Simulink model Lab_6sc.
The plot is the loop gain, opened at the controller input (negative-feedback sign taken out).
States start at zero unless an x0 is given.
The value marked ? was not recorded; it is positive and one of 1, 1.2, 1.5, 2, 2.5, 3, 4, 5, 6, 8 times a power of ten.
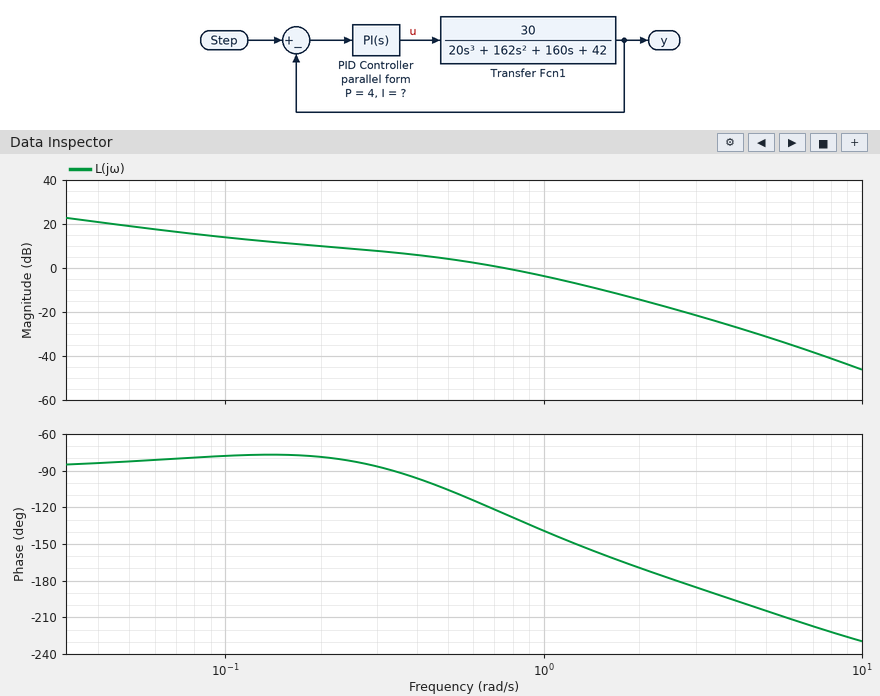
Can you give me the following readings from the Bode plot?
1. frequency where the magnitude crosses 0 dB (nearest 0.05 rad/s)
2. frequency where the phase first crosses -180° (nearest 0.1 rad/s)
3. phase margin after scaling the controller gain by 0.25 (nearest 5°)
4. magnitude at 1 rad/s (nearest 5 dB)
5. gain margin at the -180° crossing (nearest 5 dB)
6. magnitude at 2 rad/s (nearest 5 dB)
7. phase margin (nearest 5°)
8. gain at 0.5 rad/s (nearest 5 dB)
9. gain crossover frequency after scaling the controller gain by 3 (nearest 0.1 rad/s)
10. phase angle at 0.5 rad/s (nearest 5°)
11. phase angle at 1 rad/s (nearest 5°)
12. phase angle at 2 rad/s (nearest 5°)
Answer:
0.75 rad/s
2.6 rad/s
105°
-5 dB
20 dB
-15 dB
55°
5 dB
1.5 rad/s
-105°
-140°
-170°
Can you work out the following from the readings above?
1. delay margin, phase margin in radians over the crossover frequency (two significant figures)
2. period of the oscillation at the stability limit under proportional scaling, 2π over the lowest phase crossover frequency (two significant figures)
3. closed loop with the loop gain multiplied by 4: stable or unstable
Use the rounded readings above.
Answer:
1.3 s
2.4 s
stable
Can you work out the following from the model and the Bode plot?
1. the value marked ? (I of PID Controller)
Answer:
0.6
